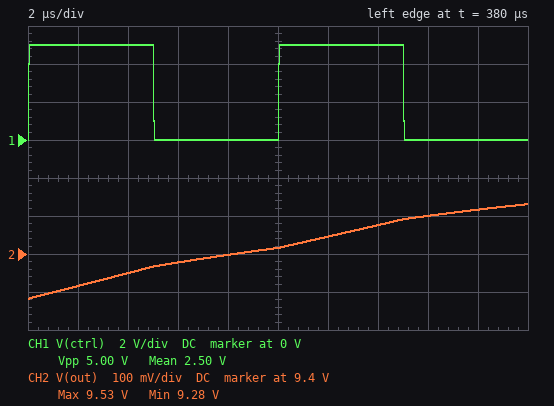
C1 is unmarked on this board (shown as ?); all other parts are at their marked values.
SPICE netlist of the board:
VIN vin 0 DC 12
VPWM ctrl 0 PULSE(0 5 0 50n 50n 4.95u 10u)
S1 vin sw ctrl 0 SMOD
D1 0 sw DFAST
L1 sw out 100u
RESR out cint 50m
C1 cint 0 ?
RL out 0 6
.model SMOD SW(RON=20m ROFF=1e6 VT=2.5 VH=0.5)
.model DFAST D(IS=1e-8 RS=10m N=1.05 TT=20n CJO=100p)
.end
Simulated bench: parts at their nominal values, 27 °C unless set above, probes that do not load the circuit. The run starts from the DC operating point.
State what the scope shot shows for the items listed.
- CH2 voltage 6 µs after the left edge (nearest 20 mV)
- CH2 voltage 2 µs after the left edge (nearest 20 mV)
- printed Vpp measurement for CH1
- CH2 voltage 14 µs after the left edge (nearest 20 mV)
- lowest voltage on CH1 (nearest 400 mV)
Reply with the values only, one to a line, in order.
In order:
9.38 V
9.32 V
5.00 V
9.48 V
0 V
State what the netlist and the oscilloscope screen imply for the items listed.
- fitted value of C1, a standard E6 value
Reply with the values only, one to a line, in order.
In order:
220 µF
